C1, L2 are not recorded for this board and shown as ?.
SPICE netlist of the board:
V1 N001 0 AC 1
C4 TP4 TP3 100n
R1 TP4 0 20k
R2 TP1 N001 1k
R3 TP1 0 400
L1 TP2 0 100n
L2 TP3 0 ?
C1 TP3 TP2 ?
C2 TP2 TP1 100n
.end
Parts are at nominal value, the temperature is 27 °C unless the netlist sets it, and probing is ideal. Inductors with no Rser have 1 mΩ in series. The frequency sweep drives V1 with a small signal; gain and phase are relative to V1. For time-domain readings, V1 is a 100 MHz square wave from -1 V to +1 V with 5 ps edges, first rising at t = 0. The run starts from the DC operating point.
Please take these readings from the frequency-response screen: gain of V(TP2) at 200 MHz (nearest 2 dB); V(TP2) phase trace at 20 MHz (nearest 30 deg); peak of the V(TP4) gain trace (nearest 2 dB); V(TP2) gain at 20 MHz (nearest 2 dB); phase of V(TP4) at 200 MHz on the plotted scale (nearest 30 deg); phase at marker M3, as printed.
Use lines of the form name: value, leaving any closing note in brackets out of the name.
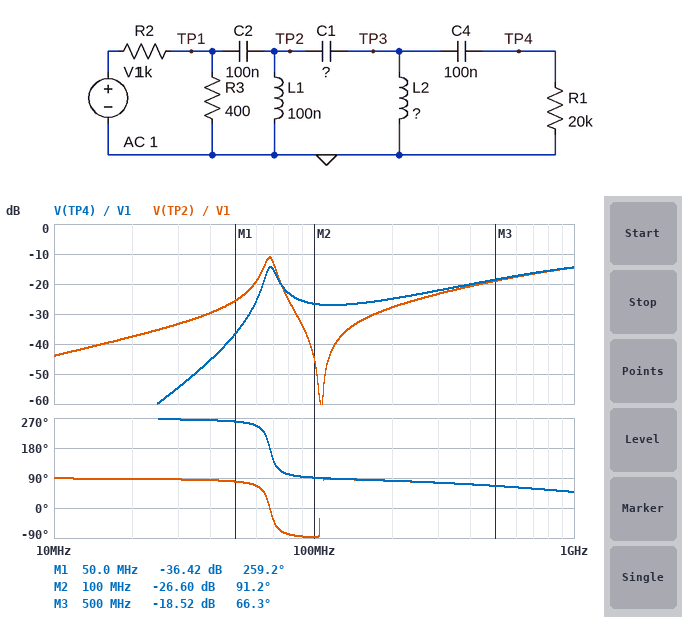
gain of V(TP2) at 200 MHz: -28 dB
V(TP2) phase trace at 20 MHz: 90 deg
peak of the V(TP4) gain trace: -14 dB
V(TP2) gain at 20 MHz: -38 dB
phase of V(TP4) at 200 MHz on the plotted scale: 90 deg
phase at marker M3, as printed: 66.3 deg
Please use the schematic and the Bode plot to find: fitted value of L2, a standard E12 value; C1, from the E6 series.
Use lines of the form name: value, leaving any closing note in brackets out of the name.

fitted value of L2, a standard E12 value: 68 nH
C1, from the E6 series: 33 pF
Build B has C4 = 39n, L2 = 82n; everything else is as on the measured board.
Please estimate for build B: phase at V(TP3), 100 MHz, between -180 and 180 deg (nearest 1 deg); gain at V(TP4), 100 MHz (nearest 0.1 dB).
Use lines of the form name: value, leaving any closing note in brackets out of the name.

phase at V(TP3), 100 MHz, between -180 and 180 deg: 89 deg
gain at V(TP4), 100 MHz: -26.2 dB
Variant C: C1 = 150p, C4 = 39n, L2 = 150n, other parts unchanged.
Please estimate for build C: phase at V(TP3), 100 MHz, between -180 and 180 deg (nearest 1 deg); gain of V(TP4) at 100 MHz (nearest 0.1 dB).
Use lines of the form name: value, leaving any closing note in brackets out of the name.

phase at V(TP3), 100 MHz, between -180 and 180 deg: 83 deg
gain of V(TP4) at 100 MHz: -27.9 dB
